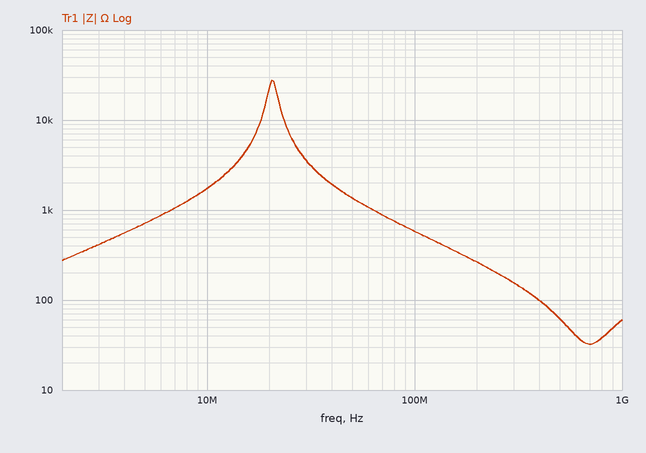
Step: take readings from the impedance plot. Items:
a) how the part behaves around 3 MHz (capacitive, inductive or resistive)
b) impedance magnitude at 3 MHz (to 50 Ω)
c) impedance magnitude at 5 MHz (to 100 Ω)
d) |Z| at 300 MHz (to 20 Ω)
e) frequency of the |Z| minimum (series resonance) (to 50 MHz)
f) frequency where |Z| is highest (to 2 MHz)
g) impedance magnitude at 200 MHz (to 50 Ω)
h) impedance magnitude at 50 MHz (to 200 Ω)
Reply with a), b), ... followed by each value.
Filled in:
a) inductive
b) 400 Ω
c) 700 Ω
d) 160 Ω
e) 700 MHz
f) 20 MHz
g) 250 Ω
h) 1.4 kΩ
